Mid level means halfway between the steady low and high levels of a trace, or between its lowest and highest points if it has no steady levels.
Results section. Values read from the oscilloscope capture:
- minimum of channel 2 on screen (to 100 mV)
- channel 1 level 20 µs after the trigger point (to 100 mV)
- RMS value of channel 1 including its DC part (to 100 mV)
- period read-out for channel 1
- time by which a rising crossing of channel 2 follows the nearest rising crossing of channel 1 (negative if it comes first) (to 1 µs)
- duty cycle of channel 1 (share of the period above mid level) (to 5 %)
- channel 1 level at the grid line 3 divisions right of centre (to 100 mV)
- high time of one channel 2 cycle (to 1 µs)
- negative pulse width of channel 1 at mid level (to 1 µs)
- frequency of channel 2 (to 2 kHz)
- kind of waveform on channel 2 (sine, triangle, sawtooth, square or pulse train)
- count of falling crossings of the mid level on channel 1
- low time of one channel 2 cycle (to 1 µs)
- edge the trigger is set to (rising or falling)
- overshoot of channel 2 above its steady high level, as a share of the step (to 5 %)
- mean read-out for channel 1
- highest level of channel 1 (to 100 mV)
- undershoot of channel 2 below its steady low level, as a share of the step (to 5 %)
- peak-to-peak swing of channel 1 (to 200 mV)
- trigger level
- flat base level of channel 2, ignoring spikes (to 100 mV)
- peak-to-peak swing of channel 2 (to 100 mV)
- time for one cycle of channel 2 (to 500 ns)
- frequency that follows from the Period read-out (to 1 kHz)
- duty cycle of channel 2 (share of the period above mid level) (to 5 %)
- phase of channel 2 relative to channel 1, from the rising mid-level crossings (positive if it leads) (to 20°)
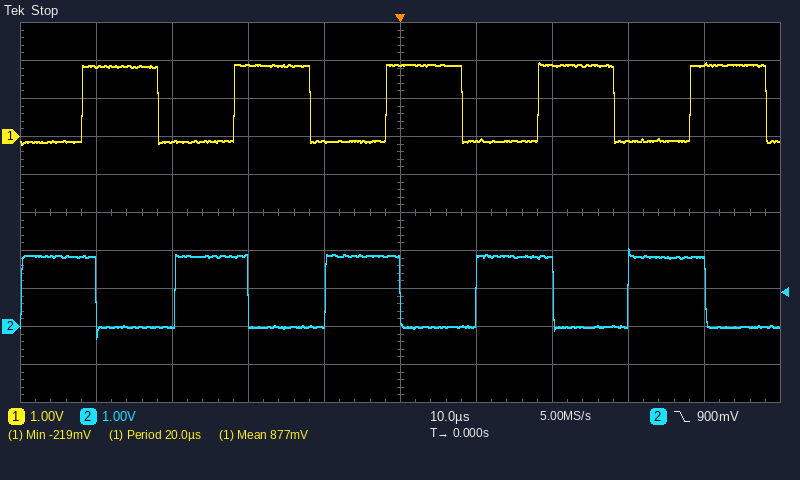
-300 mV
1.9 V
1.3 V
20.0 µs
-8 µs
50 %
-100 mV
10 µs
10 µs
50 kHz
square
5
10 µs
falling
10 %
877 mV
1.9 V
15 %
2.2 V
900 mV
0.0 V
2.4 V
20.0 µs
50 kHz
50 %
+140°
